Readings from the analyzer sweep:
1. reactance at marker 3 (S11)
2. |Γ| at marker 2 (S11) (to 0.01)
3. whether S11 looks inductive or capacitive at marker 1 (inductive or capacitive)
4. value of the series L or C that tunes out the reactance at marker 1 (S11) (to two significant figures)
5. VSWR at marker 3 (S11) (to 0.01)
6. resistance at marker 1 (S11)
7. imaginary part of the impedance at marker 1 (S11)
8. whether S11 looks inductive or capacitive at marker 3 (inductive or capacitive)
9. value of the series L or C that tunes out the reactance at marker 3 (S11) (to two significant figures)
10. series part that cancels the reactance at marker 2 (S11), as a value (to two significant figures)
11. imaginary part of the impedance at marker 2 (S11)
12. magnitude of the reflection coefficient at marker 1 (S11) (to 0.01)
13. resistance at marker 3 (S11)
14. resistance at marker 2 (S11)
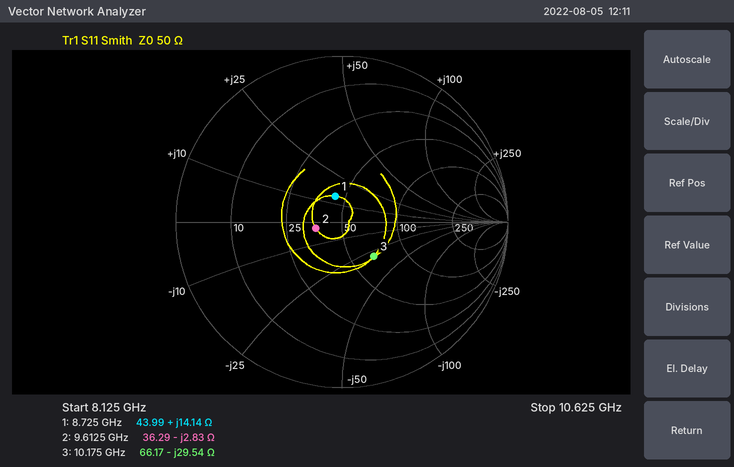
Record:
-29.54 Ω
0.16
inductive
1.3 pF
1.78
43.99 Ω
+14.14 Ω
capacitive
460 pH
47 pH
-2.83 Ω
0.16
66.17 Ω
36.29 Ω
